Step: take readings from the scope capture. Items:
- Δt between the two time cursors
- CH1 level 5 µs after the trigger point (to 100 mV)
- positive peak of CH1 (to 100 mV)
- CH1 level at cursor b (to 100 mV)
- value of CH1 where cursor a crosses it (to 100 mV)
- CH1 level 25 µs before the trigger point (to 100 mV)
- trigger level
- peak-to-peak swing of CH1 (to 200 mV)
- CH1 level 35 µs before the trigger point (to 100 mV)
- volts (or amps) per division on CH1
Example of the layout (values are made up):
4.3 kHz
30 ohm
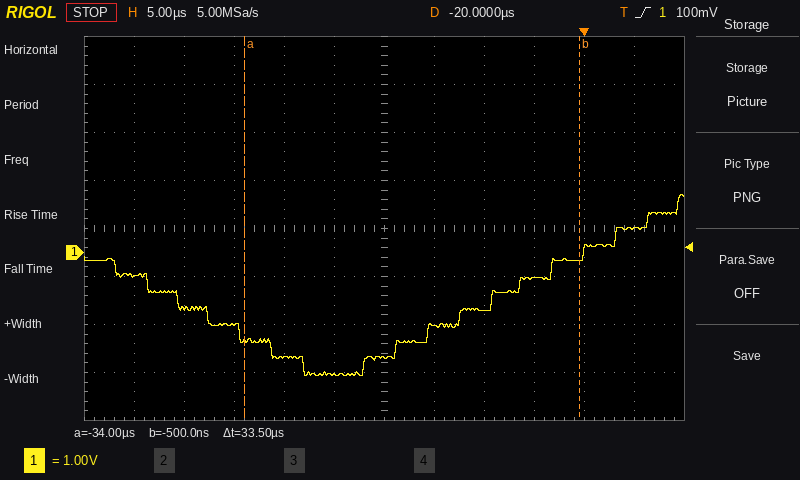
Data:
33.5 µs
500 mV
1.2 V
-100 mV
-1.8 V
-2.5 V
100 mV
3.8 V
-1.5 V
1 V
